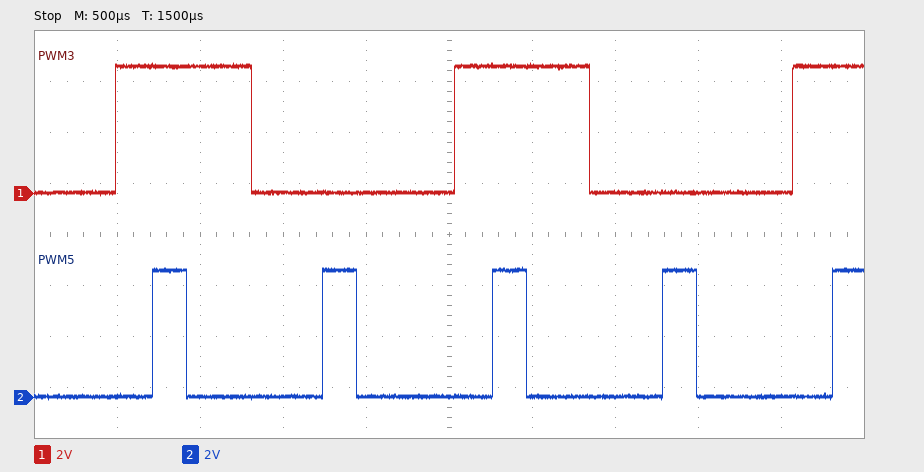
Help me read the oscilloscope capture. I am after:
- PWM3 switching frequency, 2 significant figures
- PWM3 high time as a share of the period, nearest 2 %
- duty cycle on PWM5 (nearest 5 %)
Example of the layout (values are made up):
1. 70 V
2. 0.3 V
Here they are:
1. 490 Hz
2. 40 %
3. 20 %
